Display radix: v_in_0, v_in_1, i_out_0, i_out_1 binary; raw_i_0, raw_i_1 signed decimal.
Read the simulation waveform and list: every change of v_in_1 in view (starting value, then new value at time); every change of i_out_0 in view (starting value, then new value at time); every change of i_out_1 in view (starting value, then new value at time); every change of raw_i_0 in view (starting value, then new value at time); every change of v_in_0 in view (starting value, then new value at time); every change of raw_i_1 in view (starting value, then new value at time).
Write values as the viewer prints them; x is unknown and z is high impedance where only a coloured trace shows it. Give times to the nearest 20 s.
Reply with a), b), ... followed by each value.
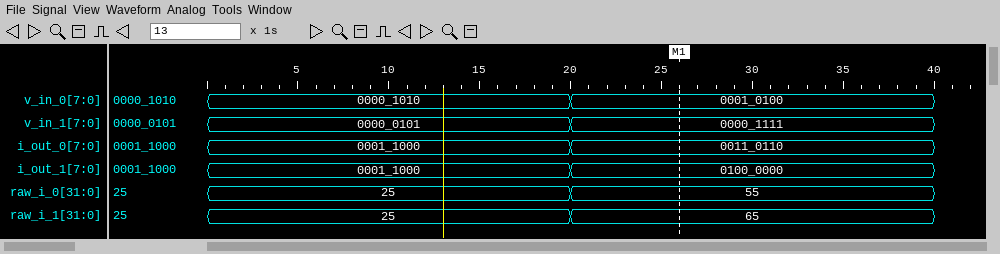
a) 0000_0101, 0000_1111 at 20 s
b) 0001_1000, 0011_0110 at 20 s
c) 0001_1000, 0100_0000 at 20 s
d) 25, 55 at 20 s
e) 0000_1010, 0001_0100 at 20 s
f) 25, 65 at 20 s
